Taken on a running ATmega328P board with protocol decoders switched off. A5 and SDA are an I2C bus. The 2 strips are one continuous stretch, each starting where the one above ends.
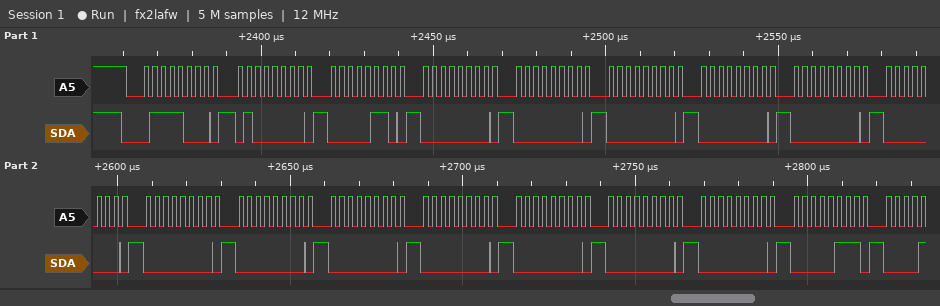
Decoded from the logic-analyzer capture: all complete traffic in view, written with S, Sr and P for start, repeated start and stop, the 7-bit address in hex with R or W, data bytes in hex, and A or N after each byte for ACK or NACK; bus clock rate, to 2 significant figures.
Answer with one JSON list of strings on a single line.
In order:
["S 3CW A 40 A 06 A 00 A 00 A 00 A 00 A 00 A 00 A 00 A 00 A 00 A 00 A 00 A 00 A 00 A 07 A", "400 kHz"]
